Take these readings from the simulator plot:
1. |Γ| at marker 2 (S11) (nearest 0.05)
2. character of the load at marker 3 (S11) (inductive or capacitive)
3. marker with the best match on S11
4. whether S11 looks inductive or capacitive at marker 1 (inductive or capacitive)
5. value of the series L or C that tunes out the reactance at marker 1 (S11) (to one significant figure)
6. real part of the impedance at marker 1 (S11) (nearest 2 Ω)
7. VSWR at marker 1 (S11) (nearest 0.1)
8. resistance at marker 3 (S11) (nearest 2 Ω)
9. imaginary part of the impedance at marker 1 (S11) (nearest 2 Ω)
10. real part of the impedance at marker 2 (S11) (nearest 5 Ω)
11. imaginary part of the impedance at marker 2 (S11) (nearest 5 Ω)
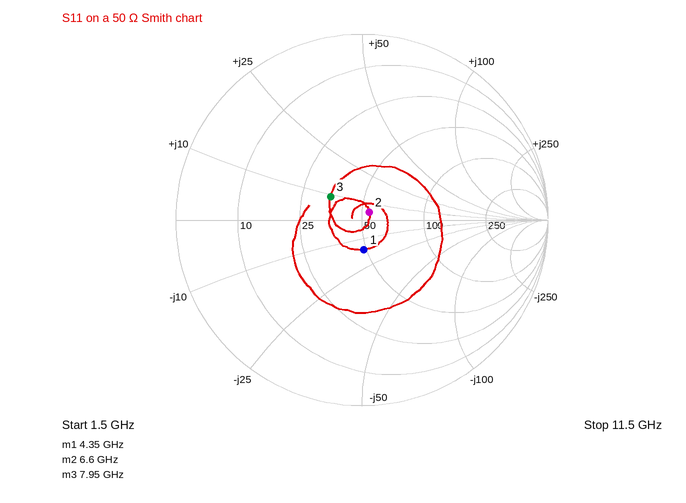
0.05
inductive
marker 2
capacitive
600 pH
48 Ω
1.4
34 Ω
-16 Ω
55 Ω
+5 Ω
